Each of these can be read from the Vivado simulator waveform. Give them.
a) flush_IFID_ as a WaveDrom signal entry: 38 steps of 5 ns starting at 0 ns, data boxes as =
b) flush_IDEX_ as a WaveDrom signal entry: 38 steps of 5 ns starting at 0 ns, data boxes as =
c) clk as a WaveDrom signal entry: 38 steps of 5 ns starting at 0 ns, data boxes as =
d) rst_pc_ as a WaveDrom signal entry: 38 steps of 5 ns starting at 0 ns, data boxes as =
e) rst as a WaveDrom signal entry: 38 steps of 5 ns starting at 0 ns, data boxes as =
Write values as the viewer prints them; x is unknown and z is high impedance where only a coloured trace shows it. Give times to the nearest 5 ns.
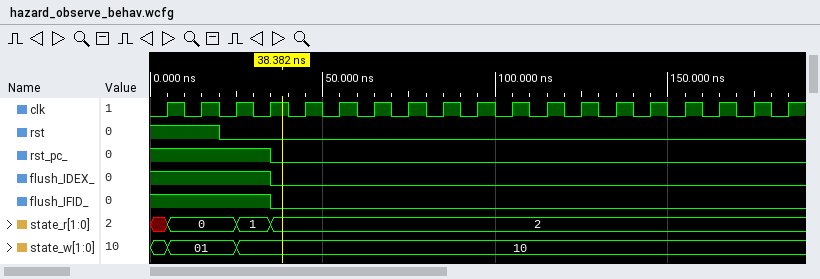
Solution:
{name: 'flush_IFID_', wave: '1......0..............................'}
{name: 'flush_IDEX_', wave: '1......0..............................'}
{name: 'clk', wave: '01010101010101010101010101010101010101'}
{name: 'rst_pc_', wave: '1......0..............................'}
{name: 'rst', wave: '1...0.................................'}
